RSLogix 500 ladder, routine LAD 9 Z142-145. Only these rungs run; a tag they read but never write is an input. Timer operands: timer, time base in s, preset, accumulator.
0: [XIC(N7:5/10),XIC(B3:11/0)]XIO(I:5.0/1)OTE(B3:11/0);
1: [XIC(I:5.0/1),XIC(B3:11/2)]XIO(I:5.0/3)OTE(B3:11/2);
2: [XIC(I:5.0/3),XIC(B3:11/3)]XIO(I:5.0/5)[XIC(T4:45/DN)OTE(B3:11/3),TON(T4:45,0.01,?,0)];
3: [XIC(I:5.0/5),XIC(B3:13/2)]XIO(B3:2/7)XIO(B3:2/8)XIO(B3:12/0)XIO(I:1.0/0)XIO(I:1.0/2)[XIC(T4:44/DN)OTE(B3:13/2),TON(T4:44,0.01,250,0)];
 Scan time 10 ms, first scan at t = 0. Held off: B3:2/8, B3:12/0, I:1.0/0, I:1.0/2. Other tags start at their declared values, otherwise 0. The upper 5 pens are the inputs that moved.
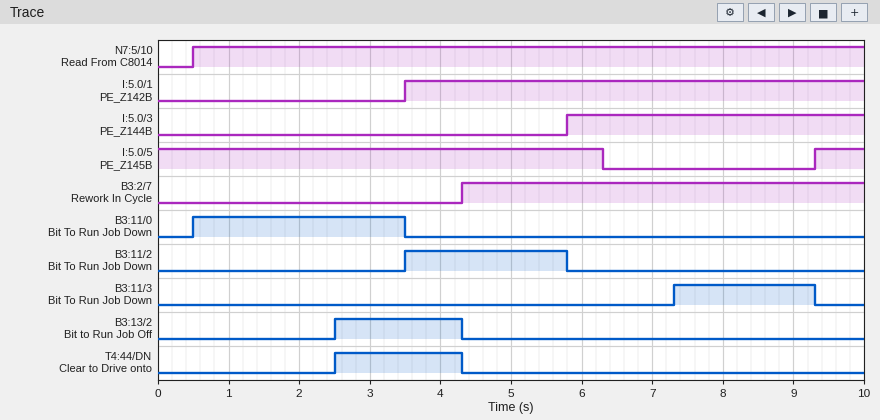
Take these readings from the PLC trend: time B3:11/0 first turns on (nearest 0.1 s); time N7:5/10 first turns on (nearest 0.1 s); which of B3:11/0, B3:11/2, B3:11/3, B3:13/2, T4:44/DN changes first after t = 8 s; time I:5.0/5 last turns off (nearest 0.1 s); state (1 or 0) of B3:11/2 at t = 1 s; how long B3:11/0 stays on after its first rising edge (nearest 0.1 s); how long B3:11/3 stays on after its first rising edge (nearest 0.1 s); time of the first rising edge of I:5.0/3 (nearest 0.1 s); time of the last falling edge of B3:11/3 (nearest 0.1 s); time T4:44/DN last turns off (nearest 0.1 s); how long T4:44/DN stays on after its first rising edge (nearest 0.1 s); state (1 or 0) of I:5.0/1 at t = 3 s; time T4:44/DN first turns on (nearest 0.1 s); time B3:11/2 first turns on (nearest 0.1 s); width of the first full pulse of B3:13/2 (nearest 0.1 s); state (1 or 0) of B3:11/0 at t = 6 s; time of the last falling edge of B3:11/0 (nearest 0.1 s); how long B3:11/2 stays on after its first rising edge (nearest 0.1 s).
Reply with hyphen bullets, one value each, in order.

- 0.5 s
- 0.5 s
- B3:11/3
- 6.3 s
- 0
- 3.0 s
- 2.0 s
- 5.8 s
- 9.3 s
- 4.3 s
- 1.8 s
- 0
- 2.5 s
- 3.5 s
- 1.8 s
- 0
- 3.5 s
- 2.3 s
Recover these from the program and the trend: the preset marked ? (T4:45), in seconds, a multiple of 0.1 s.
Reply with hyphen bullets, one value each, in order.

- 1.0 s
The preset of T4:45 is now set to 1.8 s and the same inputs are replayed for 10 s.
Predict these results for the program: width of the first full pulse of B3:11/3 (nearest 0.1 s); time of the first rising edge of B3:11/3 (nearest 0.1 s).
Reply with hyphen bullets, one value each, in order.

- 1.2 s
- 8.1 s
